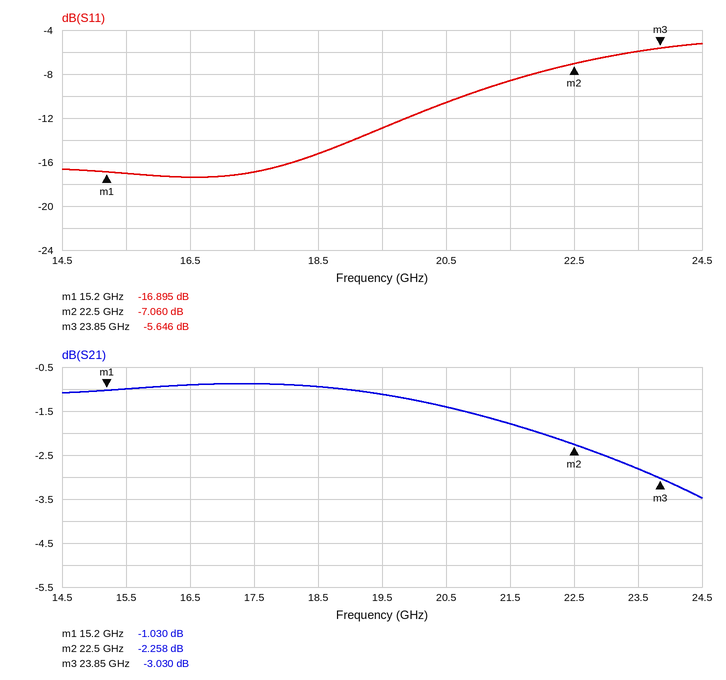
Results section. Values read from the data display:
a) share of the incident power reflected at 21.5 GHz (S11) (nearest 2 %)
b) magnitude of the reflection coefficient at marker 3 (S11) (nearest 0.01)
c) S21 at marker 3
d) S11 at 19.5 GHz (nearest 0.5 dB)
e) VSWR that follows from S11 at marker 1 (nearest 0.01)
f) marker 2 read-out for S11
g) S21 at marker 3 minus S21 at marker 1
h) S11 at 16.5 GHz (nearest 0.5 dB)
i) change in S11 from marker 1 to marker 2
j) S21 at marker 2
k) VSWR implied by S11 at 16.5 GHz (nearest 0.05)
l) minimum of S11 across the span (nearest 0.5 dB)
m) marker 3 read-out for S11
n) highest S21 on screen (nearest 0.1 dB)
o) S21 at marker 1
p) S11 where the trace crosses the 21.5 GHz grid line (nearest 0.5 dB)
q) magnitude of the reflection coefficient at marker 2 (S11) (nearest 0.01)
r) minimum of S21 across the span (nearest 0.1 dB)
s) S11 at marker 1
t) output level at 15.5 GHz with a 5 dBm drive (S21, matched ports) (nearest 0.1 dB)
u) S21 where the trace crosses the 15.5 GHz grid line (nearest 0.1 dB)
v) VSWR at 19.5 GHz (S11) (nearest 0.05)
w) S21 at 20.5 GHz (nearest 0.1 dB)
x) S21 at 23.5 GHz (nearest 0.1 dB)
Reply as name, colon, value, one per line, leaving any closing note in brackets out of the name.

share of the incident power reflected at 21.5 GHz (S11): 14 %
magnitude of the reflection coefficient at marker 3 (S11): 0.52
S21 at marker 3: -3.030 dB
S11 at 19.5 GHz: -13.0 dB
VSWR that follows from S11 at marker 1: 1.33
marker 2 read-out for S11: -7.060 dB
S21 at marker 3 minus S21 at marker 1: -2.000 dB
S11 at 16.5 GHz: -17.5 dB
change in S11 from marker 1 to marker 2: 9.835 dB
S21 at marker 2: -2.258 dB
VSWR implied by S11 at 16.5 GHz: 1.30
minimum of S11 across the span: -17.5 dB
marker 3 read-out for S11: -5.646 dB
highest S21 on screen: -0.9 dB
S21 at marker 1: -1.030 dB
S11 where the trace crosses the 21.5 GHz grid line: -8.5 dB
magnitude of the reflection coefficient at marker 2 (S11): 0.44
minimum of S21 across the span: -3.5 dB
S11 at marker 1: -16.895 dB
output level at 15.5 GHz with a 5 dBm drive (S21, matched ports): 4.0 dBm
S21 where the trace crosses the 15.5 GHz grid line: -1.0 dB
VSWR at 19.5 GHz (S11): 1.60
S21 at 20.5 GHz: -1.4 dB
S21 at 23.5 GHz: -2.8 dB
